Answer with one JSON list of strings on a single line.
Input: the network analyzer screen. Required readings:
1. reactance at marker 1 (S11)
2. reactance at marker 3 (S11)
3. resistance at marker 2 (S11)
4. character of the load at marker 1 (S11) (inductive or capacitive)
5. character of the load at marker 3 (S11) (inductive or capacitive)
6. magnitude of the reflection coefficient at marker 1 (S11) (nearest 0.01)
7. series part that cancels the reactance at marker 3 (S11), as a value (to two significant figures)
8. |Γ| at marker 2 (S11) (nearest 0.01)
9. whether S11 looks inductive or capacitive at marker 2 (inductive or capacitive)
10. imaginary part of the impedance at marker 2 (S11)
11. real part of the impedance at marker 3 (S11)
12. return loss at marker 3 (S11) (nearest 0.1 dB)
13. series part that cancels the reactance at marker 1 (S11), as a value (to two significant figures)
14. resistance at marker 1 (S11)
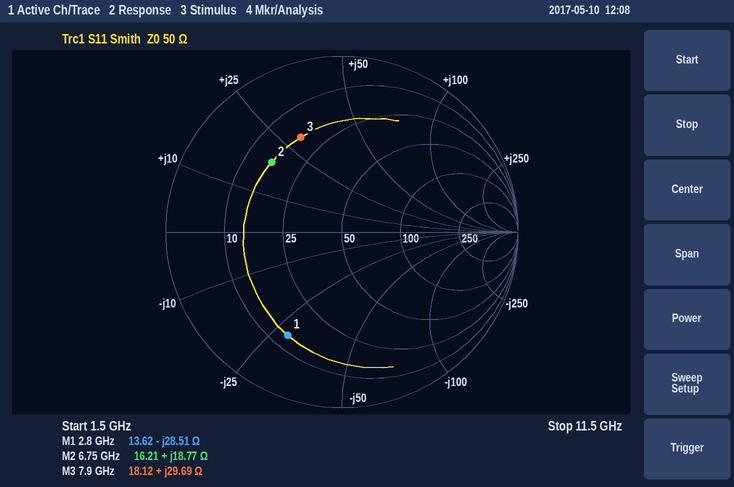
["-28.51 Ω", "+29.69 Ω", "16.21 Ω", "capacitive", "inductive", "0.66", "680 fF", "0.56", "inductive", "+18.77 Ω", "18.12 Ω", "4.6 dB", "1.6 nH", "13.62 Ω"]
